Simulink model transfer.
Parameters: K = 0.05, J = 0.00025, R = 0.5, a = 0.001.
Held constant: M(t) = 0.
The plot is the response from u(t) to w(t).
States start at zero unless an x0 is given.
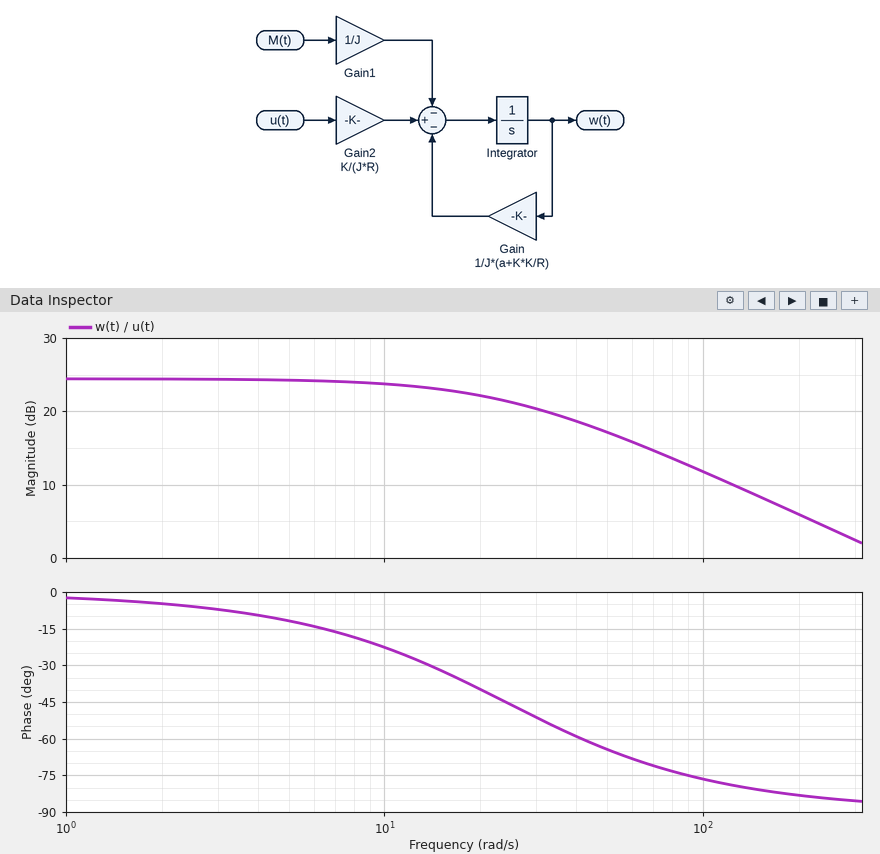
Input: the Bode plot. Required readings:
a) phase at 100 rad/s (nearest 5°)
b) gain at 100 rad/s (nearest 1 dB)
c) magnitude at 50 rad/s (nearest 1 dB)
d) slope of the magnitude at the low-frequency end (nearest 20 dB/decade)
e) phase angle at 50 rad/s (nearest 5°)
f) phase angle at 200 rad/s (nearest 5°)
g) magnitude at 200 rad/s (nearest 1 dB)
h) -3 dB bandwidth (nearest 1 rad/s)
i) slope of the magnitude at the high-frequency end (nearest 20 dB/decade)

-75°
12 dB
17 dB
0 dB/decade
-65°
-85°
6 dB
24 rad/s
-20 dB/decade
